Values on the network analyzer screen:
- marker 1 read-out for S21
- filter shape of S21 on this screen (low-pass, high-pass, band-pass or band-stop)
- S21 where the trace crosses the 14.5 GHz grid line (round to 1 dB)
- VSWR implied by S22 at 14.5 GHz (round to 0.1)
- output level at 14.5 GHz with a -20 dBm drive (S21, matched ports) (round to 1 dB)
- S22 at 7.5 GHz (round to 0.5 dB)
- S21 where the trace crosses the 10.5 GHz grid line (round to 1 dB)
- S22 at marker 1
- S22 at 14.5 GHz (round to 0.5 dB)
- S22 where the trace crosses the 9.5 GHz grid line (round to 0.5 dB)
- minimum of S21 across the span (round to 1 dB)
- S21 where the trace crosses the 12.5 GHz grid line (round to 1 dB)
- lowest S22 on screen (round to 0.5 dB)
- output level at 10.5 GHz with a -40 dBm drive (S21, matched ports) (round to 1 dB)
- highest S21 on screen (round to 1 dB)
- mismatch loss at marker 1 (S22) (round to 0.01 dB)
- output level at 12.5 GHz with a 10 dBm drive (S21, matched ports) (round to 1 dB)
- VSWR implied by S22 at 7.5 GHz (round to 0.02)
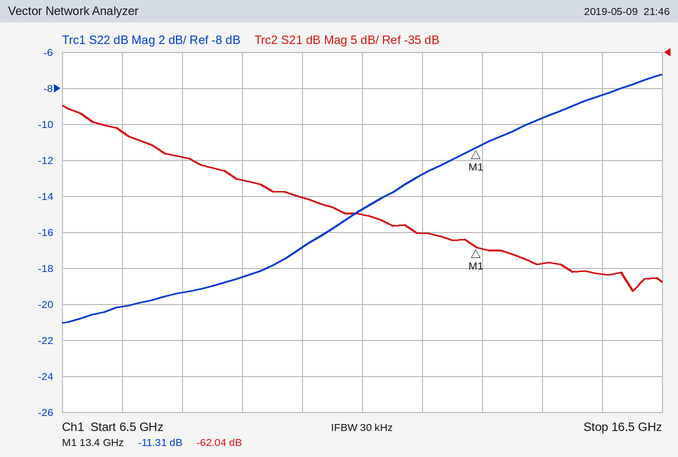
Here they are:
-62.04 dB
low-pass
-64 dB
2.0
-84 dBm
-20.0 dB
-55 dB
-11.31 dB
-9.5 dB
-18.5 dB
-68 dB
-60 dB
-21.0 dB
-95 dBm
-42 dB
0.33 dB
-50 dBm
1.22
